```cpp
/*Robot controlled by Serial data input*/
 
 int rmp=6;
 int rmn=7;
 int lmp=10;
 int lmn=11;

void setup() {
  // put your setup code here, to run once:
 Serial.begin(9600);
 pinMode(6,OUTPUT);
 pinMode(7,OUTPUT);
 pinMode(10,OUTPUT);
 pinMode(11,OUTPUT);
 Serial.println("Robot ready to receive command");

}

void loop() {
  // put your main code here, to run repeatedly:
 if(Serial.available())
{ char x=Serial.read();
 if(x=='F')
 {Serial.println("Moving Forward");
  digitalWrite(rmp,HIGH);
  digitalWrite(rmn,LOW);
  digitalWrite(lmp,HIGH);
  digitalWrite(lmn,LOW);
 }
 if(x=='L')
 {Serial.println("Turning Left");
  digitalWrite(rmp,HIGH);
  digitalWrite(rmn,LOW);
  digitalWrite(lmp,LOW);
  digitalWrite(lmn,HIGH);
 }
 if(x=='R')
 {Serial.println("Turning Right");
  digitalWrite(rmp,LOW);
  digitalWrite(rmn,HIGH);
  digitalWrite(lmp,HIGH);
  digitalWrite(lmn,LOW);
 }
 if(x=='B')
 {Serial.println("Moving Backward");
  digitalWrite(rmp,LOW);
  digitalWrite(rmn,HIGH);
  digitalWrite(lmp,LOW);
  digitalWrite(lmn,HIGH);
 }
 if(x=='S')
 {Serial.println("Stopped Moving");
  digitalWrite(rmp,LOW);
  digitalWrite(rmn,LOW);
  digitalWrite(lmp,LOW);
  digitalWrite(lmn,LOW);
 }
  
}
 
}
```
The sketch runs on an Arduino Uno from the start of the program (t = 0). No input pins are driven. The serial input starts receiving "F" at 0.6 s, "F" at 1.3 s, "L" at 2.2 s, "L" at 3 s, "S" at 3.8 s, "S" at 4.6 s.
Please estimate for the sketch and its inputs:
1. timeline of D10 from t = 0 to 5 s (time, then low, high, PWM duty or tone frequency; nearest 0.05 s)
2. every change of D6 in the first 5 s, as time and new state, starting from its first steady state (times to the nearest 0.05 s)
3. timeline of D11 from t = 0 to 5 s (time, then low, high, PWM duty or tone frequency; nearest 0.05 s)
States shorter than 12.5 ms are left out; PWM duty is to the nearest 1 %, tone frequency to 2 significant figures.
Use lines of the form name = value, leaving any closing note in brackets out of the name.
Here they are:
timeline of D10 from t = 0 to 5 s = 0 s low; 0.6 s high; 2.2 s low
every change of D6 in the first 5 s, as time and new state, starting from its first steady state = 0 s low; 0.6 s high; 3.8 s low
timeline of D11 from t = 0 to 5 s = 0 s low; 2.2 s high; 3.8 s low
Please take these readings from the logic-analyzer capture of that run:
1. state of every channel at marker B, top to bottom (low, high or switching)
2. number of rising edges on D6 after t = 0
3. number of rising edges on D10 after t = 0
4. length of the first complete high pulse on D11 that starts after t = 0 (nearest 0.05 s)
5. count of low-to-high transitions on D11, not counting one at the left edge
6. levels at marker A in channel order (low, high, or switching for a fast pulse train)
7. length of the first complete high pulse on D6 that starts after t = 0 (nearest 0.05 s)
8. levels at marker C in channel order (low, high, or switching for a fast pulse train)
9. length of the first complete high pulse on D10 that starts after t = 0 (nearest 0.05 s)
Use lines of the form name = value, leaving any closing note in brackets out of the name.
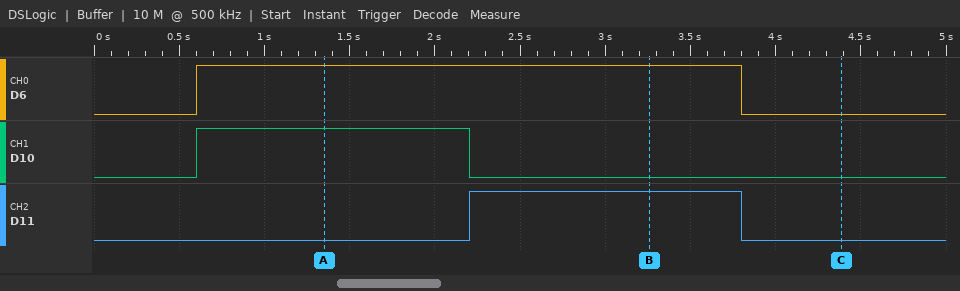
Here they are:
state of every channel at marker B, top to bottom = D6 high, D10 low, D11 high
number of rising edges on D6 after t = 0 = 1
number of rising edges on D10 after t = 0 = 1
length of the first complete high pulse on D11 that starts after t = 0 = 1.60 s
count of low-to-high transitions on D11, not counting one at the left edge = 1
levels at marker A in channel order = D6 high, D10 high, D11 low
length of the first complete high pulse on D6 that starts after t = 0 = 3.20 s
levels at marker C in channel order = D6 low, D10 low, D11 low
length of the first complete high pulse on D10 that starts after t = 0 = 1.60 s
